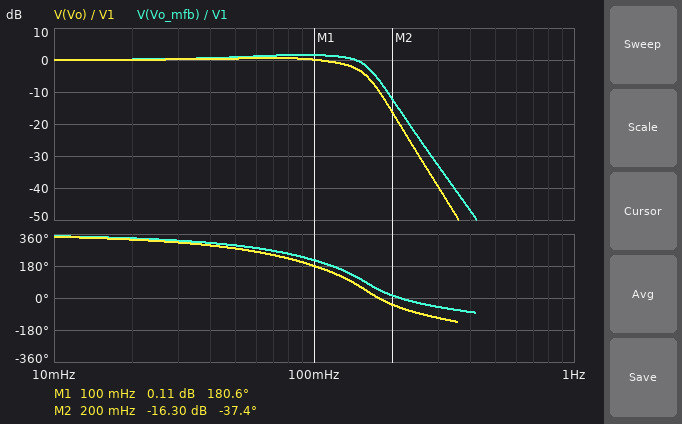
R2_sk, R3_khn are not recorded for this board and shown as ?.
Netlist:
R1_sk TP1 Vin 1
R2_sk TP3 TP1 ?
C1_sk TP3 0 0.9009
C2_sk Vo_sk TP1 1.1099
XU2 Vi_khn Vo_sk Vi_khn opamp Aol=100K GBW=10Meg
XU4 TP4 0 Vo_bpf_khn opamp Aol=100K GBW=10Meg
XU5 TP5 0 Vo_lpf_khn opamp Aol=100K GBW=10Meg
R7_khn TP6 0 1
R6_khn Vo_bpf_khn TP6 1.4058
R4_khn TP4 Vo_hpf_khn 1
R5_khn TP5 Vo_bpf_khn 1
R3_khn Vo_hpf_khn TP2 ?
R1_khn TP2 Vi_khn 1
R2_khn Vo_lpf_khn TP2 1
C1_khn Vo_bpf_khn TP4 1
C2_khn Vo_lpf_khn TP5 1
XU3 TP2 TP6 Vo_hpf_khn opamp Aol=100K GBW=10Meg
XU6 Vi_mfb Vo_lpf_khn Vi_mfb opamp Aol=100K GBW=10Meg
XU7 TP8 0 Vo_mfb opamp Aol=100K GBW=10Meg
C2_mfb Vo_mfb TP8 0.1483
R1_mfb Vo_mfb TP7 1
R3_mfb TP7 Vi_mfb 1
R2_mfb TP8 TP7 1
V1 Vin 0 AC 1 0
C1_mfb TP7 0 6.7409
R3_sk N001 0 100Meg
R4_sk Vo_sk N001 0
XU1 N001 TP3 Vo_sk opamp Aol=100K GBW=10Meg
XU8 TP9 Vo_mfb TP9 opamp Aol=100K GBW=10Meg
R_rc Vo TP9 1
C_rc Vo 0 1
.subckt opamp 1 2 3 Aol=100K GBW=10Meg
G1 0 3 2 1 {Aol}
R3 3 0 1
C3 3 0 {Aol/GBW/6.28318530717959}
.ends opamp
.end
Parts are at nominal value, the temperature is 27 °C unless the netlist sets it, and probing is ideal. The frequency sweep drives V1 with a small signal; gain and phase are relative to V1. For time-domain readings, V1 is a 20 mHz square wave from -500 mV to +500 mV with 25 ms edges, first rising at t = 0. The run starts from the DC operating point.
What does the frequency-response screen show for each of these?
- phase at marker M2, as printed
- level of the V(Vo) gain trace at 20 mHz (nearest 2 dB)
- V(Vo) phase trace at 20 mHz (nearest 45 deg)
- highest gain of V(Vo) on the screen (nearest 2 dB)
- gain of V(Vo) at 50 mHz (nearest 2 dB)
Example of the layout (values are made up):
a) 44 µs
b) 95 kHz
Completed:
a) -37.4 deg
b) 0 dB
c) 315 deg
d) 0 dB
e) 0 dB
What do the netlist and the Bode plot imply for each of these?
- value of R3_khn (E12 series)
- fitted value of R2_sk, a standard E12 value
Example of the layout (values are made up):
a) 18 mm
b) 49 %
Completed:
a) 0.47 Ω
b) 0.33 Ω
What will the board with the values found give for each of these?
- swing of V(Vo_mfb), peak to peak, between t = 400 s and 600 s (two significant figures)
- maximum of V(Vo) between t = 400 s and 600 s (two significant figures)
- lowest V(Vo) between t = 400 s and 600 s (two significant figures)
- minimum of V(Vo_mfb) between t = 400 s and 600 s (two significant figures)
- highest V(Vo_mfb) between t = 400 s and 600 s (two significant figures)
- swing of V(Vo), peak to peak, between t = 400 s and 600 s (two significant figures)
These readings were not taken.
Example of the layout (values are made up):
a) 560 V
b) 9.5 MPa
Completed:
a) 1.5 V
b) 680 mV
c) -680 mV
d) -760 mV
e) 760 mV
f) 1.4 V
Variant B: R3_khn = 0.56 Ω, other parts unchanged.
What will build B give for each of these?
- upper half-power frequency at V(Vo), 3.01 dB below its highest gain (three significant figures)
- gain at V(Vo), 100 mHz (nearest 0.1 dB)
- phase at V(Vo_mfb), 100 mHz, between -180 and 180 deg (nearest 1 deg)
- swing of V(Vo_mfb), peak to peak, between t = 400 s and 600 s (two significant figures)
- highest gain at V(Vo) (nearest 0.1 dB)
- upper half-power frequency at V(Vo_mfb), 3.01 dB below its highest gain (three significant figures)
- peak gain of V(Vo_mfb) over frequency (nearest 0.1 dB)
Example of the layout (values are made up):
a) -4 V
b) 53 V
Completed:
a) 152 mHz
b) 0.6 dB
c) -139 deg
d) 1.6 V
e) 0.7 dB
f) 161 mHz
g) 2.1 dB
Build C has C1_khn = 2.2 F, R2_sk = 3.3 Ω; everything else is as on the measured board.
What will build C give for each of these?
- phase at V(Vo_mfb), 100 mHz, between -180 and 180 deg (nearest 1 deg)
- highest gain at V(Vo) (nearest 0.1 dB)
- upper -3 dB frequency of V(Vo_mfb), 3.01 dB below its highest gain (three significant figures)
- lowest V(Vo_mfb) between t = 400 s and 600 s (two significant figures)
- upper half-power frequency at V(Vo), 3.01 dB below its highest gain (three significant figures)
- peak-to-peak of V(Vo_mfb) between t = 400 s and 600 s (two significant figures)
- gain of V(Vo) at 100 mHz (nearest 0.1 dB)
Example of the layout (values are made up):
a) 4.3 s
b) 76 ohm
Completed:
a) 110 deg
b) 0 dB
c) 80.7 mHz
d) -610 mV
e) 77.6 mHz
f) 1.2 V
g) -8.5 dB
